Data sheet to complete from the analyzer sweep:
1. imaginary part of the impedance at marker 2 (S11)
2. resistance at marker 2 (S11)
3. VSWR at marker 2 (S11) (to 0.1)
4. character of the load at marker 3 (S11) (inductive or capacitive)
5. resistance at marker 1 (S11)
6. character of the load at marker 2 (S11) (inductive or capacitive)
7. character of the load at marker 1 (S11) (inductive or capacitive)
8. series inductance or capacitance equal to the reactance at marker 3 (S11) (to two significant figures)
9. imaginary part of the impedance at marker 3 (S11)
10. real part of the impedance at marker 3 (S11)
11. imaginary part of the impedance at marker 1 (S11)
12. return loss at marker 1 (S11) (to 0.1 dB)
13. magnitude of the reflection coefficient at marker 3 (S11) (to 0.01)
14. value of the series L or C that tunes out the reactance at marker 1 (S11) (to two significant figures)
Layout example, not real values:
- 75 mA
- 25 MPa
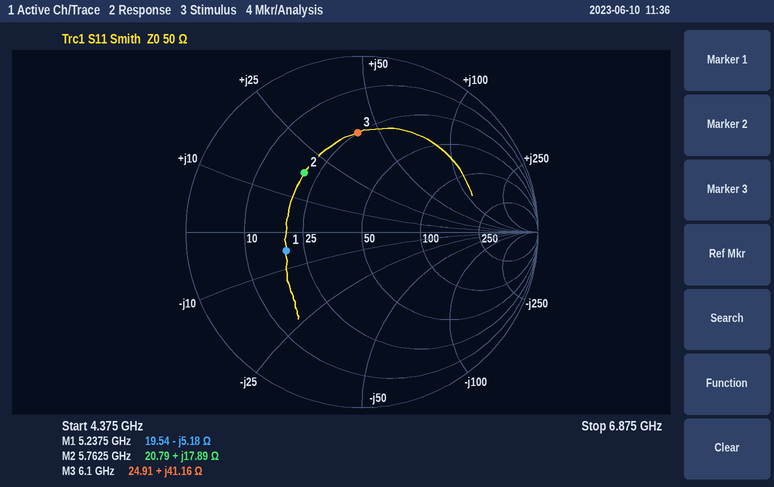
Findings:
- +17.89 Ω
- 20.79 Ω
- 2.8
- inductive
- 19.54 Ω
- inductive
- capacitive
- 1.1 nH
- +41.16 Ω
- 24.91 Ω
- -5.18 Ω
- 7.1 dB
- 0.56
- 160 pH
